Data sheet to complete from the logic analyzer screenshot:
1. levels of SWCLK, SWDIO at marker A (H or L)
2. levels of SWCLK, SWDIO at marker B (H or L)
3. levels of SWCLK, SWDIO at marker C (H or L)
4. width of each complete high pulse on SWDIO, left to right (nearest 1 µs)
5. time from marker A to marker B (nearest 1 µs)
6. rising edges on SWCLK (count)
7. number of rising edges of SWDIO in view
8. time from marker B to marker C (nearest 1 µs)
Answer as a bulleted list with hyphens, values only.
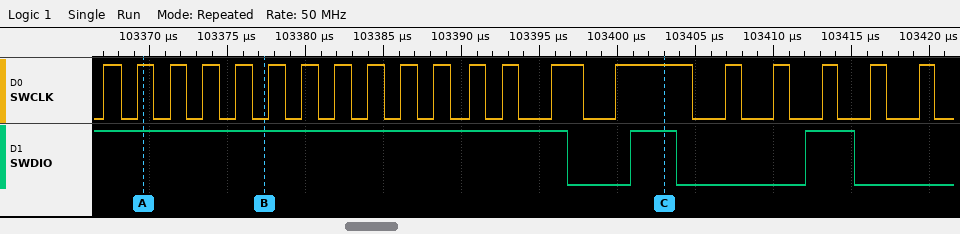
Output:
- SWCLK=H, SWDIO=H
- SWCLK=L, SWDIO=H
- SWCLK=H, SWDIO=H
- 3 µs, 3 µs
- 8 µs
- 20
- 2
- 26 µs
